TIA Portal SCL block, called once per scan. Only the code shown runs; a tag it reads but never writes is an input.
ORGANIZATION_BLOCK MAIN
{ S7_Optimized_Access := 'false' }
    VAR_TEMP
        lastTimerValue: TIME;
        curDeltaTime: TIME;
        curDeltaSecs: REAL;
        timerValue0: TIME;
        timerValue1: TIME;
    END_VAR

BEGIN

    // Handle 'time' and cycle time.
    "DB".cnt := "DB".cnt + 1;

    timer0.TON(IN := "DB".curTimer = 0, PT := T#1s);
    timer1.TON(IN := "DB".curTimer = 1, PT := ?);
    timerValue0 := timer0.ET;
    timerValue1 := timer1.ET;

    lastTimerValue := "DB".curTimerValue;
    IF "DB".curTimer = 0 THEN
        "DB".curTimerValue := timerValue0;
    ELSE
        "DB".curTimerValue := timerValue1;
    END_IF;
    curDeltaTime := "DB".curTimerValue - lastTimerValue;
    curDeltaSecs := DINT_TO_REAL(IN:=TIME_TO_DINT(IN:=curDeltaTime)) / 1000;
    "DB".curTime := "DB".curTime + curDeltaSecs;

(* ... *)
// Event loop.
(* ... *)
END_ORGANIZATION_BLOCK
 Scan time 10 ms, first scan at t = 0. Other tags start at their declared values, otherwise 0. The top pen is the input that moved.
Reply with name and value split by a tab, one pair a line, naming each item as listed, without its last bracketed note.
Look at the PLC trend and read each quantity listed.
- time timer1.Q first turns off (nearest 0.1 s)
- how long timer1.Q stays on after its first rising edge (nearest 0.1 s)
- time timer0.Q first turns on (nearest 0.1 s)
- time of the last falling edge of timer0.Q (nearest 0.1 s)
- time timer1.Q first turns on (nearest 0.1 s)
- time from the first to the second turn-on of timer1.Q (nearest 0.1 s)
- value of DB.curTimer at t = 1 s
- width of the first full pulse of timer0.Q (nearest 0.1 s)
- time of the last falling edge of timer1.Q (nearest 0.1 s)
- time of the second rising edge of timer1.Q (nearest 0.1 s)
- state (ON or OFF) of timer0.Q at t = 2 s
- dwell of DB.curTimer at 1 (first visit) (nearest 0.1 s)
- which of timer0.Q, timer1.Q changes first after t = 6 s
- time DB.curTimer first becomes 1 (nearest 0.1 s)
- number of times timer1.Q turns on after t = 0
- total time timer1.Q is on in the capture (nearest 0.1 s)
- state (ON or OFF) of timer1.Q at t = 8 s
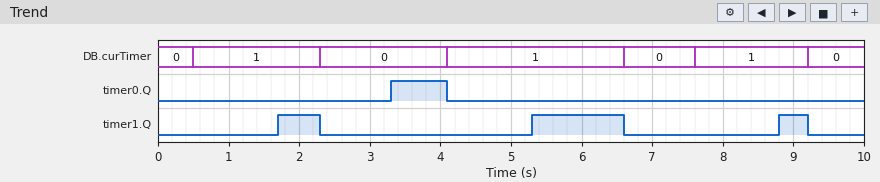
time timer1.Q first turns off	2.3 s
how long timer1.Q stays on after its first rising edge	0.6 s
time timer0.Q first turns on	3.3 s
time of the last falling edge of timer0.Q	4.1 s
time timer1.Q first turns on	1.7 s
time from the first to the second turn-on of timer1.Q	3.6 s
value of DB.curTimer at t = 1 s	1
width of the first full pulse of timer0.Q	0.8 s
time of the last falling edge of timer1.Q	9.2 s
time of the second rising edge of timer1.Q	5.3 s
state (ON or OFF) of timer0.Q at t = 2 s	OFF
dwell of DB.curTimer at 1 (first visit)	1.8 s
which of timer0.Q, timer1.Q changes first after t = 6 s	timer1.Q
time DB.curTimer first becomes 1	0.5 s
number of times timer1.Q turns on after t = 0	3
total time timer1.Q is on in the capture	2.3 s
state (ON or OFF) of timer1.Q at t = 8 s	OFF
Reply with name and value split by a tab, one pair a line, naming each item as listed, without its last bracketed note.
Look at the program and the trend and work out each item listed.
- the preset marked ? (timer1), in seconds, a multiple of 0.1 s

the preset marked ? (timer1), in seconds, a multiple of 0.1 s	1.2 s
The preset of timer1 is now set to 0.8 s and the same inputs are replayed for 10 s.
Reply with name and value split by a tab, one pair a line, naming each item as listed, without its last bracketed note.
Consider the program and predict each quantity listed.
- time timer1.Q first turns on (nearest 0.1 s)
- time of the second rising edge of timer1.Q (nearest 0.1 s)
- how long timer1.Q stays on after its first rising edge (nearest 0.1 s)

time timer1.Q first turns on	1.3 s
time of the second rising edge of timer1.Q	4.9 s
how long timer1.Q stays on after its first rising edge	1.0 s
